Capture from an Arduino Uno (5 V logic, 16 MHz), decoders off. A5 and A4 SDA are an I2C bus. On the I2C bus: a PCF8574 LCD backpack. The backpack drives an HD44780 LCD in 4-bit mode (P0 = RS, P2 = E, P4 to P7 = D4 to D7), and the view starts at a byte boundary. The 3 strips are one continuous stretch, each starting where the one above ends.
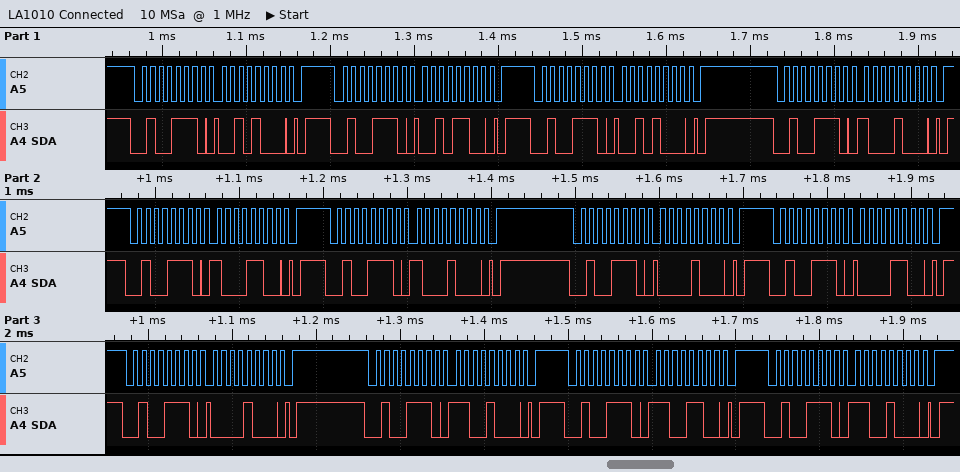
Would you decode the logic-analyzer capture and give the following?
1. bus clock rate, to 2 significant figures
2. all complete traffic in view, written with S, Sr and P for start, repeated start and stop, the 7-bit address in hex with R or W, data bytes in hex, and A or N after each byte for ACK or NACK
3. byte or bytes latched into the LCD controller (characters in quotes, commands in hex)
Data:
100 kHz
S 27W A 28 A P S 27W A 2C A P S 27W A 28 A P S 27W A 88 A P S 27W A 8C A P S 27W A 88 A P S 27W A 08 A P S 27W A 0C A P S 27W A 08 A P S 27W A C8 A P S 27W A CC A P S 27W A C8 A P
0x28 0x0C
